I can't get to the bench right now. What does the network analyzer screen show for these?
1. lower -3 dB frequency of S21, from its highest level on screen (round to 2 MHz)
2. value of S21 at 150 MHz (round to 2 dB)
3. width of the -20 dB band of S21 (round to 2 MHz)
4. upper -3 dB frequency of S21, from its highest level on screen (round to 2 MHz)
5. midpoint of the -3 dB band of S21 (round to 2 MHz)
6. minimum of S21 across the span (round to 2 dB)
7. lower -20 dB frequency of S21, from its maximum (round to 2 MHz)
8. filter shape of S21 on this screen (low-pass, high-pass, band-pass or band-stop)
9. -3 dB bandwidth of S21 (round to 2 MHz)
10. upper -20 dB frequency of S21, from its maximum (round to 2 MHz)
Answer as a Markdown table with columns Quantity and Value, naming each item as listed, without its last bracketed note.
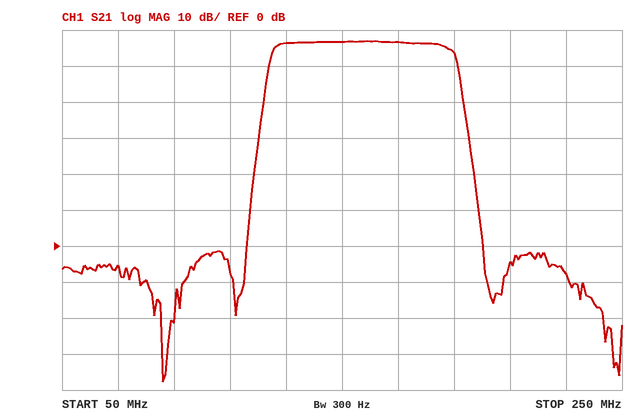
| Quantity | Value |
|---|---|
| lower -3 dB frequency of S21, from its highest level on screen | 126 MHz |
| value of S21 at 150 MHz | 56 dB |
| width of the -20 dB band of S21 | 72 MHz |
| upper -3 dB frequency of S21, from its highest level on screen | 190 MHz |
| midpoint of the -3 dB band of S21 | 158 MHz |
| minimum of S21 across the span | -38 dB |
| lower -20 dB frequency of S21, from its maximum | 122 MHz |
| filter shape of S21 on this screen | band-pass |
| -3 dB bandwidth of S21 | 64 MHz |
| upper -20 dB frequency of S21, from its maximum | 194 MHz |
